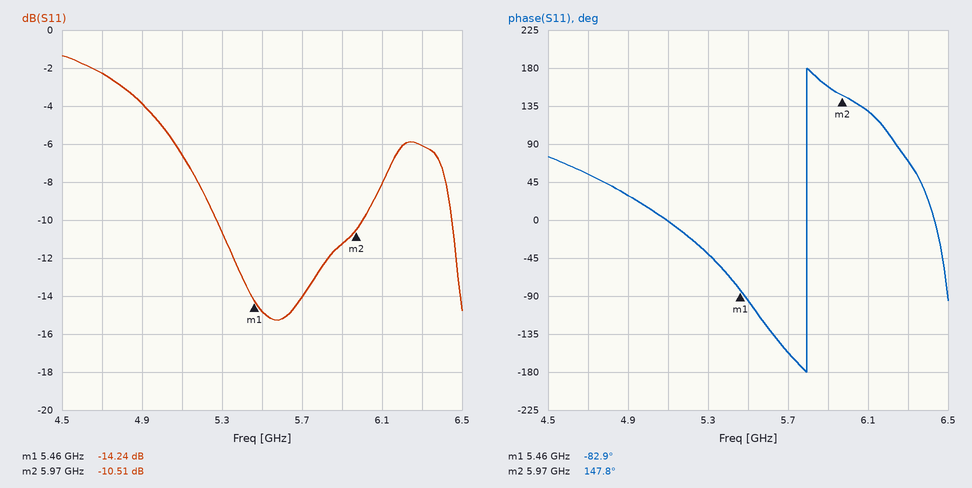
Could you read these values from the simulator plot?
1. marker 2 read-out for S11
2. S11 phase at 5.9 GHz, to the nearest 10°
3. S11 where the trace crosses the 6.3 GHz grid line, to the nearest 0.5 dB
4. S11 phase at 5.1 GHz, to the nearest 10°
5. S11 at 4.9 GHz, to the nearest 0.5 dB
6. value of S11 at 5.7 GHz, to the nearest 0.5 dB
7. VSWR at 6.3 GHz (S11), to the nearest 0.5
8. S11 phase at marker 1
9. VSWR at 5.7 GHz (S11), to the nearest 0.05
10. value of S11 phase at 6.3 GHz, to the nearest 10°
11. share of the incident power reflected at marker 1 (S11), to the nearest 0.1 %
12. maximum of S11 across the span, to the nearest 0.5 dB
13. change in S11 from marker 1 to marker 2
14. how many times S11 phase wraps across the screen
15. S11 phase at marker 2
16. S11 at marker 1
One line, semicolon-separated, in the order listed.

-10.51 dB; 160°; -6.0 dB; 0°; -4.0 dB; -14.0 dB; 3.0; -82.9°; 1.50; 70°; 3.8 %; -1.5 dB; 3.73 dB; 1; 147.8°; -14.24 dB
